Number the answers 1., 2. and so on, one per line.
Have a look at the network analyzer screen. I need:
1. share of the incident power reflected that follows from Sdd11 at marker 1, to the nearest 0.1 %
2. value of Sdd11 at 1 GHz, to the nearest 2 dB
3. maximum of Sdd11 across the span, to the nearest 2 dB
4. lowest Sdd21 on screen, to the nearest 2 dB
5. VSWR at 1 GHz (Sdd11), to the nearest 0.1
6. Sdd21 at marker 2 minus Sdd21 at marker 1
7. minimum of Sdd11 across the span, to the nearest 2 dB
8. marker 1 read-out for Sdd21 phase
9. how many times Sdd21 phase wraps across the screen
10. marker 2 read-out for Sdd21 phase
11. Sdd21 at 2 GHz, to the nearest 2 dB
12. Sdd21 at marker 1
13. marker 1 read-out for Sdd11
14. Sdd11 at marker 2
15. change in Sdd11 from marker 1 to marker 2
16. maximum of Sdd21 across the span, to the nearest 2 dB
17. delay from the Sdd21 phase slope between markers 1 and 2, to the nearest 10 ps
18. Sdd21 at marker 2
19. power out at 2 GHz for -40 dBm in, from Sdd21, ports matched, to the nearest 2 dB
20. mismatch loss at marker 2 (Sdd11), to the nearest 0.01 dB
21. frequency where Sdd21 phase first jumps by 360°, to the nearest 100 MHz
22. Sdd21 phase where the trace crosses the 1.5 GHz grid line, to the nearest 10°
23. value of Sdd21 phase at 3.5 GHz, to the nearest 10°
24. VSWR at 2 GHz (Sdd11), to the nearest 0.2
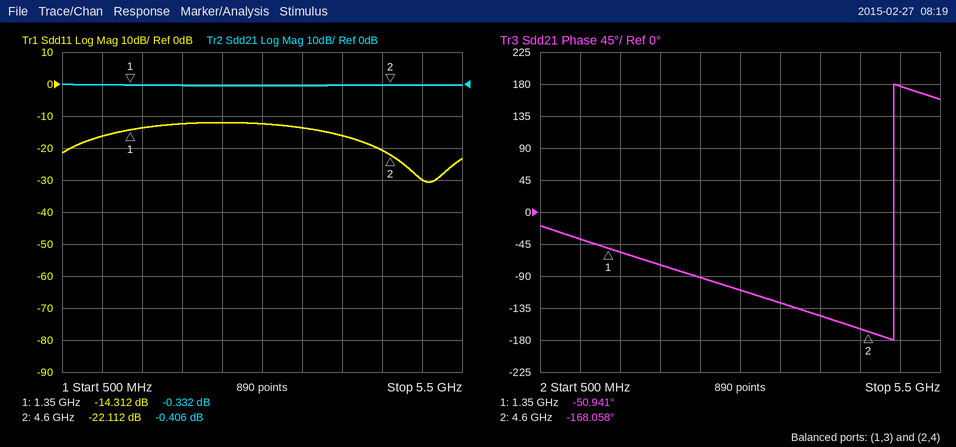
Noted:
1. 3.7 %
2. -16 dB
3. -12 dB
4. 0 dB
5. 1.4
6. -0.074 dB
7. -30 dB
8. -50.941°
9. 1
10. -168.058°
11. 0 dB
12. -0.332 dB
13. -14.312 dB
14. -22.112 dB
15. -7.800 dB
16. 0 dB
17. 100 ps
18. -0.406 dB
19. -40 dBm
20. 0.03 dB
21. 4.9 GHz
22. -60°
23. -130°
24. 1.6
